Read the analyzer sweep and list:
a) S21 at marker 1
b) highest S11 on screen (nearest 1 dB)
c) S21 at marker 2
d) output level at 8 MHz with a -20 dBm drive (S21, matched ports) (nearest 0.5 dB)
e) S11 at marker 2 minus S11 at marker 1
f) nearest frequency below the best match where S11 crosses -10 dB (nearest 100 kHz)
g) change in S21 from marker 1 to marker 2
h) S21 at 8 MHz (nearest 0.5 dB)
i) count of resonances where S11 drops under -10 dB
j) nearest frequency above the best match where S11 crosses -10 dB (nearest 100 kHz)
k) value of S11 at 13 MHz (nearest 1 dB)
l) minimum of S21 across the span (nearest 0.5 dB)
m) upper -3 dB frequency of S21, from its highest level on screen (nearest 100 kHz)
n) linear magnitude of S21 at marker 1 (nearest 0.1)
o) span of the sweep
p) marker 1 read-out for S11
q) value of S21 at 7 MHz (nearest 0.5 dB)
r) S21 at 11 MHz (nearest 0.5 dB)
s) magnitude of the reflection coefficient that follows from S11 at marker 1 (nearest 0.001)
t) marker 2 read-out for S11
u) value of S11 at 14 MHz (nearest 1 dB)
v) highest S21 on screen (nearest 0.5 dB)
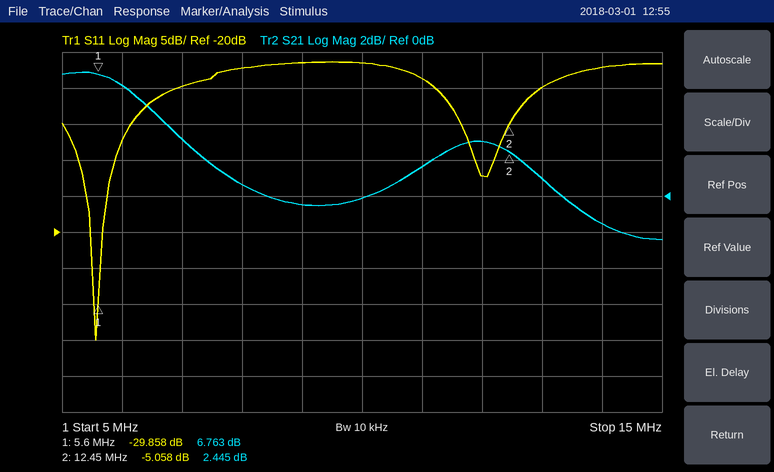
6.763 dB
4 dB
2.445 dB
-19.5 dBm
24.800 dB
5.3 MHz
-4.318 dB
0.5 dB
2
5.9 MHz
0 dB
-2.5 dB
6.8 MHz
2.2
10 MHz
-29.858 dB
3.0 dB
1.5 dB
0.032
-5.058 dB
3 dB
7.0 dB
